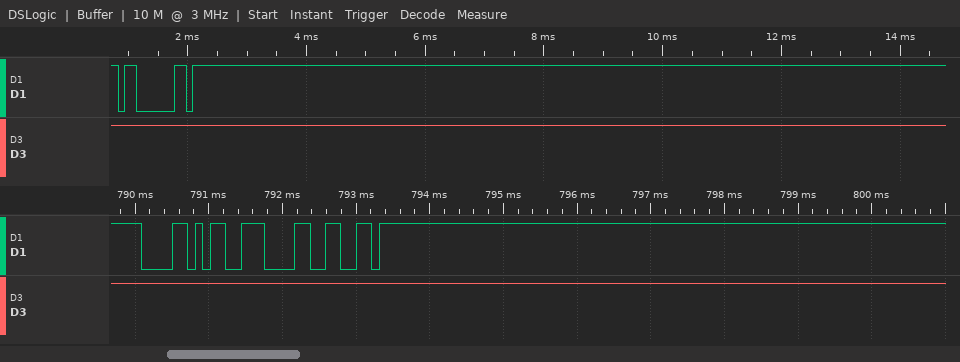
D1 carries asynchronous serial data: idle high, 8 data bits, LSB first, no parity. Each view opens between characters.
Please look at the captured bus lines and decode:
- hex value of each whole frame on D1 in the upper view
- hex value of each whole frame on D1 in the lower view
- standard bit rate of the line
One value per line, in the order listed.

03, FF
58, 0E, 66
9600 baud
